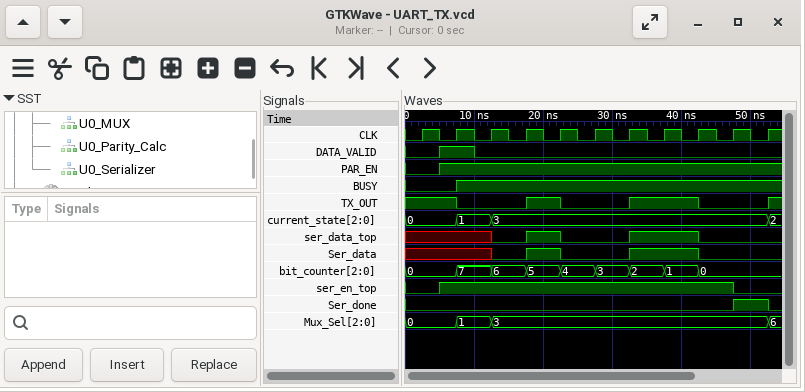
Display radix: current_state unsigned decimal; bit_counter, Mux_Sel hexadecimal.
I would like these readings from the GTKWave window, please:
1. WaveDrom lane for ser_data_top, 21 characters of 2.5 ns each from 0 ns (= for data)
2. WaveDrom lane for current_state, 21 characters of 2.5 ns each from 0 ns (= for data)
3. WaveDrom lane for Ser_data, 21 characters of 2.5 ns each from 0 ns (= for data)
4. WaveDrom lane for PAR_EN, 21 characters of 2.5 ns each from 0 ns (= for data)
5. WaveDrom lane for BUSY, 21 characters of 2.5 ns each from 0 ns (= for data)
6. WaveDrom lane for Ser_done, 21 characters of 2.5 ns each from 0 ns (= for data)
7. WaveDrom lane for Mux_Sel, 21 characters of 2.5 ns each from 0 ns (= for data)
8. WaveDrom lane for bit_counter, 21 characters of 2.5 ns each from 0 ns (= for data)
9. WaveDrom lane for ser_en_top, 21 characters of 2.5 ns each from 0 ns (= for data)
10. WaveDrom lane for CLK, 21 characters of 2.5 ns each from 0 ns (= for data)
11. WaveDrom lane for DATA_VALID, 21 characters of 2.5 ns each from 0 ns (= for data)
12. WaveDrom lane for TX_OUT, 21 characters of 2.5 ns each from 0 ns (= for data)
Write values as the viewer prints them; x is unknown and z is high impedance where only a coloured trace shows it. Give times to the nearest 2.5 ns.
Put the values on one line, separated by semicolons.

{name: 'ser_data_top', wave: 'x....0.1.0...1...0...'}; {name: 'current_state', wave: '=..=.=...............', data: '0 1 3'}; {name: 'Ser_data', wave: 'x....0.1.0...1...0...'}; {name: 'PAR_EN', wave: '0.1..................'}; {name: 'BUSY', wave: '0..1.................'}; {name: 'Ser_done', wave: '0..................1.'}; {name: 'Mux_Sel', wave: '=..=.=...............', data: '0 1 3'}; {name: 'bit_counter', wave: '=..=.=.=.=.=.=.=.=...', data: '0 7 6 5 4 3 2 1 0'}; {name: 'ser_en_top', wave: '0.1................0.'}; {name: 'CLK', wave: '010101010101010101010'}; {name: 'DATA_VALID', wave: '0.1.0................'}; {name: 'TX_OUT', wave: '1..0...1.0...1...0...'}
